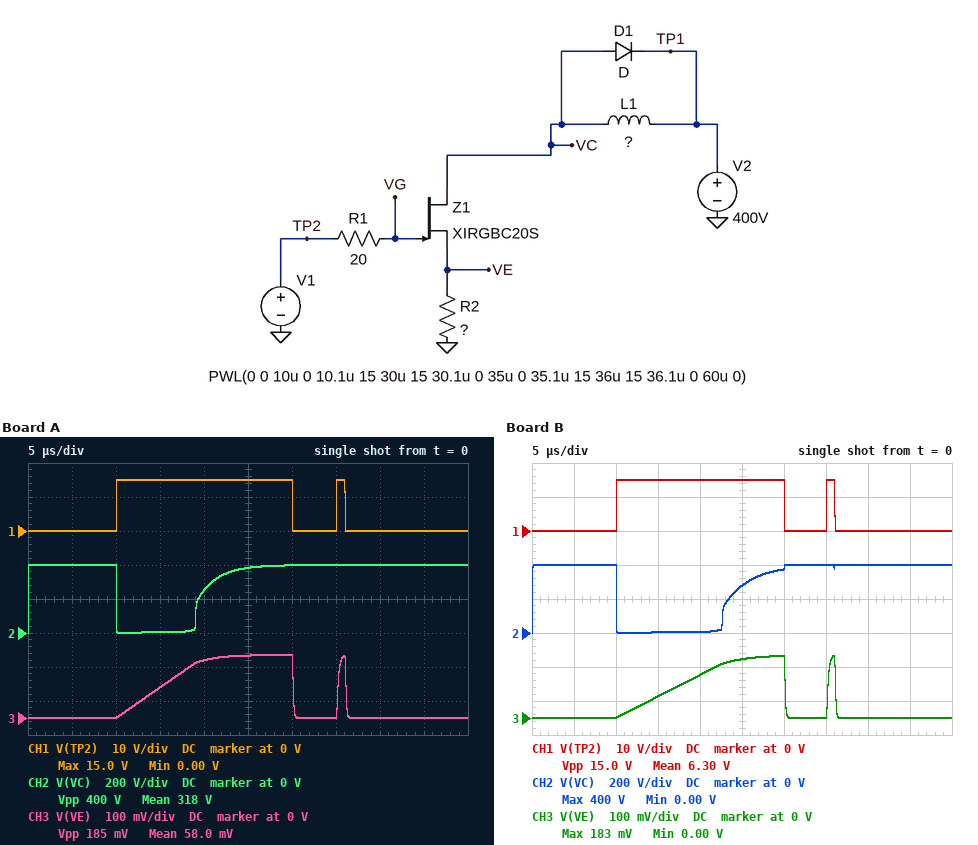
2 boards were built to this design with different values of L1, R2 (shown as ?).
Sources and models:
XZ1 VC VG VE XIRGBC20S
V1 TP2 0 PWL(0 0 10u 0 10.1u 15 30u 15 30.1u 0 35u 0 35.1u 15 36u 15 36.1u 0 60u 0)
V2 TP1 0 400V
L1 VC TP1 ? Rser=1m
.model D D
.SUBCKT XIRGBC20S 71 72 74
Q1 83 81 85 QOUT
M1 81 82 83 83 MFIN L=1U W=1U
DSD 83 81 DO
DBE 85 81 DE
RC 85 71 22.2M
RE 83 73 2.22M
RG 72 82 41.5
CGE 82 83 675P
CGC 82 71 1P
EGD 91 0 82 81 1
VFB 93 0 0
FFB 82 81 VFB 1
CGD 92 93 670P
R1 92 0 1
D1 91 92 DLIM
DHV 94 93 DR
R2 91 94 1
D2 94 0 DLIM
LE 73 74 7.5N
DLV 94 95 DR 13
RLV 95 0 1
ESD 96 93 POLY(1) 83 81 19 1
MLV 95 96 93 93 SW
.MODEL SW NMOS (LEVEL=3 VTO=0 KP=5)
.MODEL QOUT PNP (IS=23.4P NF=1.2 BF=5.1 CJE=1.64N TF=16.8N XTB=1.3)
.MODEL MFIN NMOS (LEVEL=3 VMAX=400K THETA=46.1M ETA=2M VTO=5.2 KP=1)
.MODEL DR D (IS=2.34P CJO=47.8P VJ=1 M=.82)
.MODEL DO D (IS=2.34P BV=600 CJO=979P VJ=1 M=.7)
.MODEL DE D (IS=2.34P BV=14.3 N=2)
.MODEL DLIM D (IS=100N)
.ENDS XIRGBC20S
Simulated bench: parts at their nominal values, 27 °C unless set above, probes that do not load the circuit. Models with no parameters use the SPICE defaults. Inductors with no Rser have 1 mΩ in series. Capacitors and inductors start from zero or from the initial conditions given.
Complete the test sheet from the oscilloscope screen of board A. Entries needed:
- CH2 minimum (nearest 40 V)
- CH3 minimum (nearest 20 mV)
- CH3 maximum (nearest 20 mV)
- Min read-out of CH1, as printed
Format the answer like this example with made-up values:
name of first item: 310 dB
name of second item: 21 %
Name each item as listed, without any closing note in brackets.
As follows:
CH2 minimum: 0 V
CH3 minimum: 0 V
CH3 maximum: 180 mV
Min read-out of CH1, as printed: 0.00 V
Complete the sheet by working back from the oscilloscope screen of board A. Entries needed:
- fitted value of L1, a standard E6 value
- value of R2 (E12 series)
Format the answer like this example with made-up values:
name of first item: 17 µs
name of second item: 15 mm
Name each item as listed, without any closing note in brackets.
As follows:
fitted value of L1, a standard E6 value: 33 µH
value of R2: 1.5 mΩ
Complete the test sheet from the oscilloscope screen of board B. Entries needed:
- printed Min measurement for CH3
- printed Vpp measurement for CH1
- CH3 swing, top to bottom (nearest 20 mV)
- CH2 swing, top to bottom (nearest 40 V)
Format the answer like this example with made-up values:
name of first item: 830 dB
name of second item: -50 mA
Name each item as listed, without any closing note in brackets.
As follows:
printed Min measurement for CH3: 0.00 V
printed Vpp measurement for CH1: 15.0 V
CH3 swing, top to bottom: 180 mV
CH2 swing, top to bottom: 400 V
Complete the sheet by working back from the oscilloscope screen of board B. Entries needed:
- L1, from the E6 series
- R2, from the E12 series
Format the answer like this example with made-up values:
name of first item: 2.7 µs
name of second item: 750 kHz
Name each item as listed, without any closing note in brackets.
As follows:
L1, from the E6 series: 47 µH
R2, from the E12 series: 1.5 mΩ
